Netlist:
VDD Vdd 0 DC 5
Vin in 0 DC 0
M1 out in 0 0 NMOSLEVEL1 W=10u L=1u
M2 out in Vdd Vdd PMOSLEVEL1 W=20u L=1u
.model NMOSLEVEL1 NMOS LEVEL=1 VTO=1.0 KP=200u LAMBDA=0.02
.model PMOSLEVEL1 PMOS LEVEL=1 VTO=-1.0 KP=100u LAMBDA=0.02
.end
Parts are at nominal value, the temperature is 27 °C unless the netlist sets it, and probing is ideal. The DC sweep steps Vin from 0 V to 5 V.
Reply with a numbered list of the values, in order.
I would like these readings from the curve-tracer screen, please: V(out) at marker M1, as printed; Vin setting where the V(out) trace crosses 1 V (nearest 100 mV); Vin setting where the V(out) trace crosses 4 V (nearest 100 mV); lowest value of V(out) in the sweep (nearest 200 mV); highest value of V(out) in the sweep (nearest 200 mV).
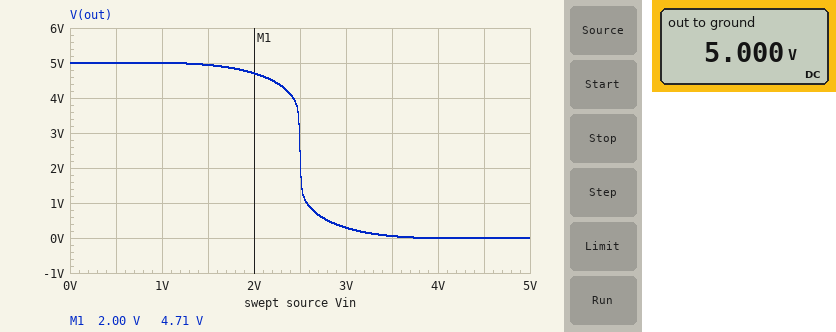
1. 4.71 V
2. 2.6 V
3. 2.4 V
4. 0 V
5. 5.0 V
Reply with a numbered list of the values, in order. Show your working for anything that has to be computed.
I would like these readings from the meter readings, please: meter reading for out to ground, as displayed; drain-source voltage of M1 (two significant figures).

1. 5.000 V
2. 5 V = 5.0 V
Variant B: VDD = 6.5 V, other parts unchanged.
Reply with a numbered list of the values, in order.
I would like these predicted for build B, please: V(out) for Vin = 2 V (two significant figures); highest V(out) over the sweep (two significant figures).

1. 6.3 V
2. 6.5 V
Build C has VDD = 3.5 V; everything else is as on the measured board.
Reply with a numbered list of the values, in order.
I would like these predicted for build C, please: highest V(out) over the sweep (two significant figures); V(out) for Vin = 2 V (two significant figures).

1. 3.5 V
2. 140 mV
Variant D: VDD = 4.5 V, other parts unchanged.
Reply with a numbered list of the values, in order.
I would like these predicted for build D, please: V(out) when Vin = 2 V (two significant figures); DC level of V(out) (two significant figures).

1. 4.1 V
2. 4.5 V
